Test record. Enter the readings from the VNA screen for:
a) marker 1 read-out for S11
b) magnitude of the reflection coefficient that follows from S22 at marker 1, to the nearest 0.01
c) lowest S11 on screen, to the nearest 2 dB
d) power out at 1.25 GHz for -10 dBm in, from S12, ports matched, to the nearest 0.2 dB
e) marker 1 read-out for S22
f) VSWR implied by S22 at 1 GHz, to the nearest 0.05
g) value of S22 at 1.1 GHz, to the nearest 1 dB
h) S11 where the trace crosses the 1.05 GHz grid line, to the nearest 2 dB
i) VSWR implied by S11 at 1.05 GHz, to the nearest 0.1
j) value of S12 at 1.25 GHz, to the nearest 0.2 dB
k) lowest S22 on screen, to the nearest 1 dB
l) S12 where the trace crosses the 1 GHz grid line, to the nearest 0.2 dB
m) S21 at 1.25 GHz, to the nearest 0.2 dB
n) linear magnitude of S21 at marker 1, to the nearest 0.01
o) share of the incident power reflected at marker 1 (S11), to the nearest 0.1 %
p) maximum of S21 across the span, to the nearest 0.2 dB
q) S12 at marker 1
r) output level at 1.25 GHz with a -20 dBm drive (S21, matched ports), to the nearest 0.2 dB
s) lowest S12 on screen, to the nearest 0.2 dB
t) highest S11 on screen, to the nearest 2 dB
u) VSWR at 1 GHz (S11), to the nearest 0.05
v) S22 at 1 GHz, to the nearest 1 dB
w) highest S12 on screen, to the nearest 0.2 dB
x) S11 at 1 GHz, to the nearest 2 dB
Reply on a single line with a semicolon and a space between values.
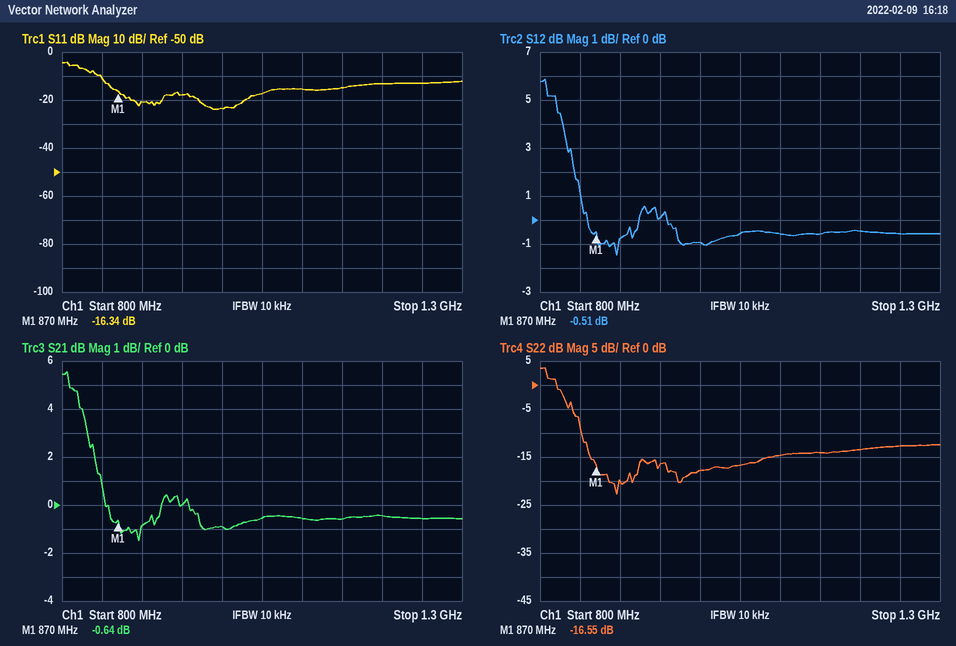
-16.34 dB; 0.15; -24 dB; -10.6 dBm; -16.55 dB; 1.30; -15 dB; -18 dB; 1.3; -0.6 dB; -23 dB; -1.0 dB; -0.6 dB; 0.93; 2.3 %; 5.6 dB; -0.51 dB; -20.6 dBm; -1.4 dB; -4 dB; 1.15; -18 dB; 5.8 dB; -24 dB
